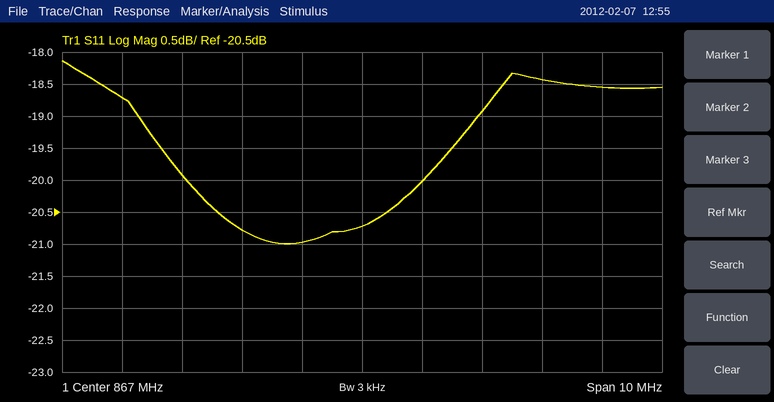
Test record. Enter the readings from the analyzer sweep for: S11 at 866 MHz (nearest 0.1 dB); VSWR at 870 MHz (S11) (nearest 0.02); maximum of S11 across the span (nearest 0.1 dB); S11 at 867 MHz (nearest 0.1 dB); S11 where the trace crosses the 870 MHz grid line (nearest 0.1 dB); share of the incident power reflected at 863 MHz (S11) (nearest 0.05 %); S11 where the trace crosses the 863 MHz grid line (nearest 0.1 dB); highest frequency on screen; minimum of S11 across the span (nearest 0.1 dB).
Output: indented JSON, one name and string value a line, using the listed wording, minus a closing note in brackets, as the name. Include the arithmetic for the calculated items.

{
  "S11 at 866 MHz": "-21.0 dB",
  "VSWR at 870 MHz (S11)": "|Γ| = 10^(-18.4/20) = 0.1202; VSWR = (1 + 0.1202)/(1 − 0.1202) ≈ 1.27, so 1.28 to the nearest 0.02",
  "maximum of S11 across the span": "-18.1 dB",
  "S11 at 867 MHz": "-20.7 dB",
  "S11 where the trace crosses the 870 MHz grid line": "-18.4 dB",
  "share of the incident power reflected at 863 MHz (S11)": "10^(-18.7/10) ≈ 1.35 %",
  "S11 where the trace crosses the 863 MHz grid line": "-18.7 dB",
  "highest frequency on screen": "872 MHz",
  "minimum of S11 across the span": "-21.0 dB"
}
